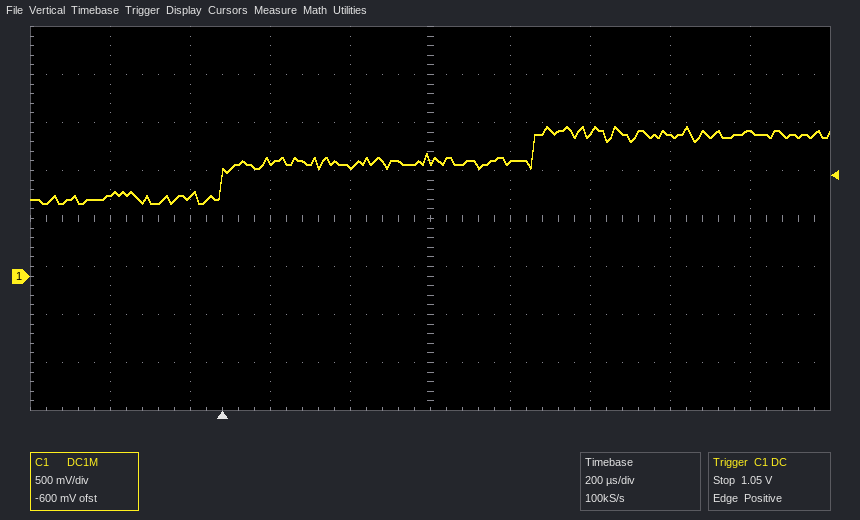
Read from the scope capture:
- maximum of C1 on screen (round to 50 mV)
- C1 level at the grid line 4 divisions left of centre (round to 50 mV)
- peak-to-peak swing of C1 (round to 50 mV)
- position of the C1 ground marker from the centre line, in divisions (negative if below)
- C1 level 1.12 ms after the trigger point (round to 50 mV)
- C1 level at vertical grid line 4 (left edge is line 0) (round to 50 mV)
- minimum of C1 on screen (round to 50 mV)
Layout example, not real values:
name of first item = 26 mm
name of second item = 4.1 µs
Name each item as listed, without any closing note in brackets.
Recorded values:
maximum of C1 on screen = 1.55 V
C1 level at the grid line 4 divisions left of centre = 850 mV
peak-to-peak swing of C1 = 800 mV
position of the C1 ground marker from the centre line, in divisions = -1.2 div
C1 level 1.12 ms after the trigger point = 1.45 V
C1 level at vertical grid line 4 (left edge is line 0) = 1.15 V
minimum of C1 on screen = 750 mV
